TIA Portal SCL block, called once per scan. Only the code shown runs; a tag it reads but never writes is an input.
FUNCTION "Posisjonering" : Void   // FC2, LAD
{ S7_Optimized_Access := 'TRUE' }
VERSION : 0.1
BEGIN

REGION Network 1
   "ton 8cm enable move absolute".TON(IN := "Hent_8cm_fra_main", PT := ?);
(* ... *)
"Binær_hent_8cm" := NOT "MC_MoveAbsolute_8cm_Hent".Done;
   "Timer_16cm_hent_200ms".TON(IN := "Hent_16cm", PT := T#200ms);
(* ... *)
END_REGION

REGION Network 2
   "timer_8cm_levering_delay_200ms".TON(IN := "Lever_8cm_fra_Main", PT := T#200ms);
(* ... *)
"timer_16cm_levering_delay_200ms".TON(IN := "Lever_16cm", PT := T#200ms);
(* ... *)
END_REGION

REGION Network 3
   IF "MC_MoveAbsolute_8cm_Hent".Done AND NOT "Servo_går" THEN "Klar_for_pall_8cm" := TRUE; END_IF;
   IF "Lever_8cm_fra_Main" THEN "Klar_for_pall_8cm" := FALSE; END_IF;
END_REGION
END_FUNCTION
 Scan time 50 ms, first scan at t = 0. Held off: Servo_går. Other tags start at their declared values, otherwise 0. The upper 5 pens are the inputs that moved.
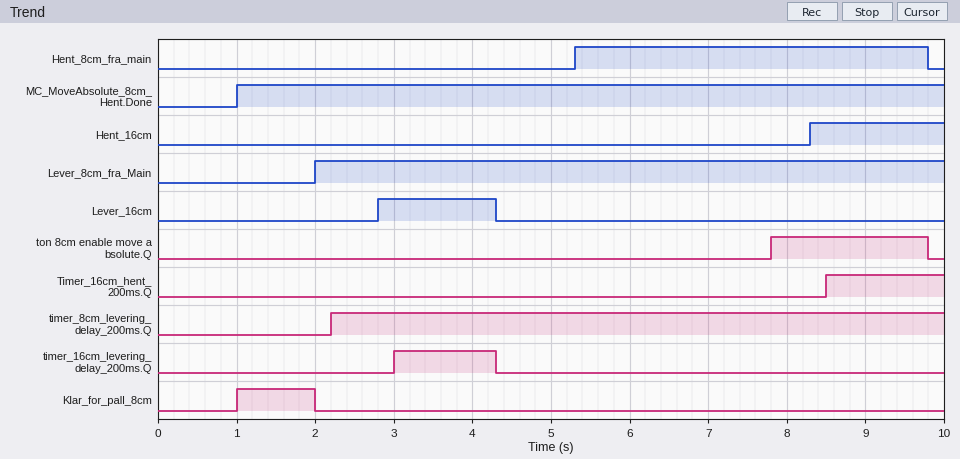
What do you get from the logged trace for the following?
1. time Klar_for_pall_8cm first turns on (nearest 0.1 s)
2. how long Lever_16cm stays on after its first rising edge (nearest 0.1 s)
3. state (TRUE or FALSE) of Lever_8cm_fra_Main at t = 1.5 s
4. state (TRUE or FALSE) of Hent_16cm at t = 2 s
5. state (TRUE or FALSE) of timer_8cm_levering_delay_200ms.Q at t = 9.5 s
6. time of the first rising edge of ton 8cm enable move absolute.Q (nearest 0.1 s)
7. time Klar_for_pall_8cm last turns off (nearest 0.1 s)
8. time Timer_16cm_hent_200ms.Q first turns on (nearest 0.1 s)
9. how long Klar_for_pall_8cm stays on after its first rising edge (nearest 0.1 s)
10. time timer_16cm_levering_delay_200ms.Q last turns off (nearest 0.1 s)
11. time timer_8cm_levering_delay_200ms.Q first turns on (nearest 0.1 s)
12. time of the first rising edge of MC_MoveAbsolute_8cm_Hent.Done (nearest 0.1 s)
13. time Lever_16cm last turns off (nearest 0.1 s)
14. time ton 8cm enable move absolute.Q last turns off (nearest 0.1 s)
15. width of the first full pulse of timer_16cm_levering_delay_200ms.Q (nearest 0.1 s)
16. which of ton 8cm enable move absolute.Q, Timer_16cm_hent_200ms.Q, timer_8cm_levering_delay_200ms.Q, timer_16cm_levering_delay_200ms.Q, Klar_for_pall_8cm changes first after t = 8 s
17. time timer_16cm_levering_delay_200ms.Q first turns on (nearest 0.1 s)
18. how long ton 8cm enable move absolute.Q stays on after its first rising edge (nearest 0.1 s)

1.0 s
1.5 s
FALSE
FALSE
TRUE
7.8 s
2.0 s
8.5 s
1.0 s
4.3 s
2.2 s
1.0 s
4.3 s
9.8 s
1.3 s
Timer_16cm_hent_200ms.Q
3.0 s
2.0 s
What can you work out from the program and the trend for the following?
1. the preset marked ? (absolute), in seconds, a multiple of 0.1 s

2.5 s
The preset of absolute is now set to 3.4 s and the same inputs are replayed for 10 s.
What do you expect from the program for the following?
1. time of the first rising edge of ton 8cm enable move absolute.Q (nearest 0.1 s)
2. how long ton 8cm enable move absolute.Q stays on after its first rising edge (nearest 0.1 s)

8.7 s
1.1 s
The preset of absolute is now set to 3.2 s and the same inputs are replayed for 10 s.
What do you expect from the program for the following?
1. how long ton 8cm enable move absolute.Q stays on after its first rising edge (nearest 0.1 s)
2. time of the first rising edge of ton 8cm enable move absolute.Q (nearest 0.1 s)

1.3 s
8.5 s
